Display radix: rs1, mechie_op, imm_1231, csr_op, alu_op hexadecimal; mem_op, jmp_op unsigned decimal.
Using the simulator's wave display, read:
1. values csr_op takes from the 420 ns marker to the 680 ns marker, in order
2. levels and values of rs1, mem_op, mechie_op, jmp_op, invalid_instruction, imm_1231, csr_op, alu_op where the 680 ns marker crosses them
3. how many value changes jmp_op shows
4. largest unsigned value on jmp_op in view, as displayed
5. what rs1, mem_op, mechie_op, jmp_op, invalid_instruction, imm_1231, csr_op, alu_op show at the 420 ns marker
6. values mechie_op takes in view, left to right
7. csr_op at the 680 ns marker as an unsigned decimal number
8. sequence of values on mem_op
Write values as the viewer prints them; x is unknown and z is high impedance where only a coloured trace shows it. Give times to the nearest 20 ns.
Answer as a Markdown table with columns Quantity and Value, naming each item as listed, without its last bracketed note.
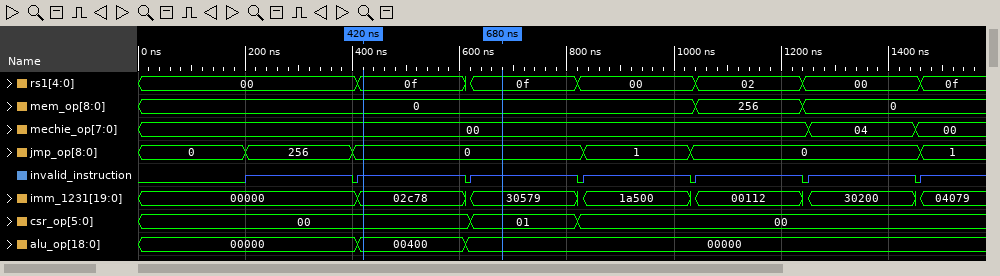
| Quantity | Value |
|---|---|
| values csr_op takes from the 420 ns marker to the 680 ns marker, in order | 00, 01 |
| levels and values of rs1, mem_op, mechie_op, jmp_op, invalid_instruction, imm_1231, csr_op, alu_op where the 680 ns marker crosses them | rs1=0f, mem_op=0, mechie_op=00, jmp_op=0, invalid_instruction=z, imm_1231=30579, csr_op=01, alu_op=00000 |
| how many value changes jmp_op shows | 5 |
| largest unsigned value on jmp_op in view, as displayed | 256 |
| what rs1, mem_op, mechie_op, jmp_op, invalid_instruction, imm_1231, csr_op, alu_op show at the 420 ns marker | rs1=0f, mem_op=0, mechie_op=00, jmp_op=0, invalid_instruction=z, imm_1231=02c78, csr_op=00, alu_op=00400 |
| values mechie_op takes in view, left to right | 00, 04, 00 |
| csr_op at the 680 ns marker as an unsigned decimal number | 1 |
| sequence of values on mem_op | 0, 256, 0 |
